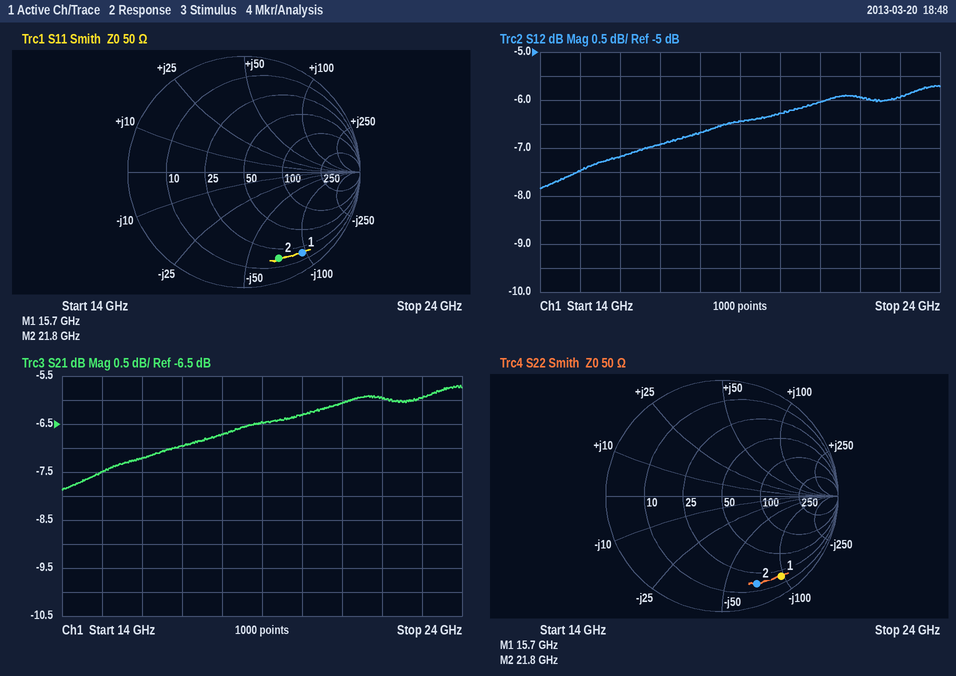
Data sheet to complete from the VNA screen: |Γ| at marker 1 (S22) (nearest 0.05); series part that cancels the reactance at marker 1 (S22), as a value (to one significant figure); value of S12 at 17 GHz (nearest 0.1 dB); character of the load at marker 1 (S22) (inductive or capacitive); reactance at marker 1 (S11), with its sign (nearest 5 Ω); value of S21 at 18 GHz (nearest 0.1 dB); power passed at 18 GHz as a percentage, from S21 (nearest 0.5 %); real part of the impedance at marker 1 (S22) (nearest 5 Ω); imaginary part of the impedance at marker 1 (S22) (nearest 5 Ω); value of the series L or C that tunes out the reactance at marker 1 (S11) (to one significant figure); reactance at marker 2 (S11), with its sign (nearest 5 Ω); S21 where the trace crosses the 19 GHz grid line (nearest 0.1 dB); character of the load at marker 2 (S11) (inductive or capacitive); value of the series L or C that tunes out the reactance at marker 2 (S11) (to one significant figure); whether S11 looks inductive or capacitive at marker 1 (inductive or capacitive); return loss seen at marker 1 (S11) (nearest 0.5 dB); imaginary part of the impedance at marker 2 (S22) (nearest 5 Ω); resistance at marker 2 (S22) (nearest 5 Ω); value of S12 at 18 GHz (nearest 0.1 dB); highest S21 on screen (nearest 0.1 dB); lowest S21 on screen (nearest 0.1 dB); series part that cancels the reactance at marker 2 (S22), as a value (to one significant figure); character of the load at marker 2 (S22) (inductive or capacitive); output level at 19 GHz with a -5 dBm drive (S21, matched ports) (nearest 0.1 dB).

0.85
1.0 nH
-6.9 dB
capacitive
-95 Ω
-6.7 dB
21.5 %
20 Ω
-95 Ω
1.0 nH
-70 Ω
-6.5 dB
capacitive
500 pH
capacitive
1.5 dB
-70 Ω
15 Ω
-6.7 dB
-5.7 dB
-7.9 dB
500 pH
capacitive
-11.5 dBm
